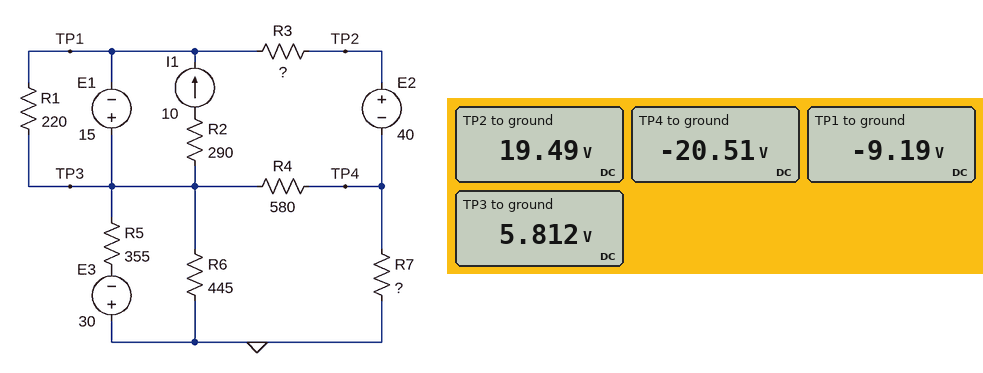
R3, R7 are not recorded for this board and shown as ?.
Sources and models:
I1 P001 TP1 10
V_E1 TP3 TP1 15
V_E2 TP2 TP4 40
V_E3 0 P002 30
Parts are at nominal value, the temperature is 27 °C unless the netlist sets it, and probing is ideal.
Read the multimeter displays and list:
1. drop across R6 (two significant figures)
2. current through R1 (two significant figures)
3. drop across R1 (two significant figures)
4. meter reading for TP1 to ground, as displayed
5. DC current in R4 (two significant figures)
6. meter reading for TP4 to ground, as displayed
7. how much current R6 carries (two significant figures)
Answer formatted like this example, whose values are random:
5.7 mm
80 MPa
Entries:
5.8 V
68 mA
15 V
-9.19 V
45 mA
-20.51 V
13 mA
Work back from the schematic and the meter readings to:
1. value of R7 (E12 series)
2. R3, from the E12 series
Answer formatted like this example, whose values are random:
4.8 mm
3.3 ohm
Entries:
180 Ω
180 Ω
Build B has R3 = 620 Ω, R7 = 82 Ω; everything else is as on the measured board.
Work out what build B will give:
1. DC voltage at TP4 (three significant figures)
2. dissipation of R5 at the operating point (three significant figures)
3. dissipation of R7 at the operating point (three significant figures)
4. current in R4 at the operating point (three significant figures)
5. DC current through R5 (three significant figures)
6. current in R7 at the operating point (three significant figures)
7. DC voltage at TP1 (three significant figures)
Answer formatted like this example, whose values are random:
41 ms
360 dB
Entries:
-6.13 V
2.22 W
458 mW
7.23 mA
79.1 mA
74.7 mA
-16.9 V
